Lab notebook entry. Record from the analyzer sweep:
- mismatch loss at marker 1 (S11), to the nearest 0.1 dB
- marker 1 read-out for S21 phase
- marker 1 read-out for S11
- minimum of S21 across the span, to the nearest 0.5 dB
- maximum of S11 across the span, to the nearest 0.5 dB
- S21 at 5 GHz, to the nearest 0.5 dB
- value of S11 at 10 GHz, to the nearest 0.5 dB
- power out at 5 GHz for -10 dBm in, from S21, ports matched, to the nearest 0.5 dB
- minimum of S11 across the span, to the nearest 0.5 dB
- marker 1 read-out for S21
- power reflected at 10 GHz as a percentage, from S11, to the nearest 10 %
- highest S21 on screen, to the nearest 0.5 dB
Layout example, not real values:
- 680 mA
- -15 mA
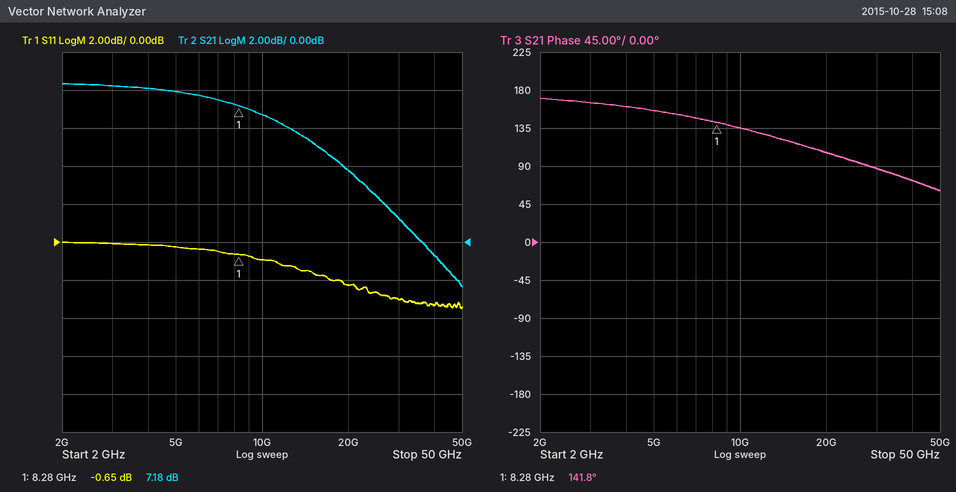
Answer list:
- 8.6 dB
- 141.8°
- -0.65 dB
- -2.5 dB
- 0.0 dB
- 8.0 dB
- -1.0 dB
- -2.0 dBm
- -3.5 dB
- 7.18 dB
- 80 %
- 8.5 dB
